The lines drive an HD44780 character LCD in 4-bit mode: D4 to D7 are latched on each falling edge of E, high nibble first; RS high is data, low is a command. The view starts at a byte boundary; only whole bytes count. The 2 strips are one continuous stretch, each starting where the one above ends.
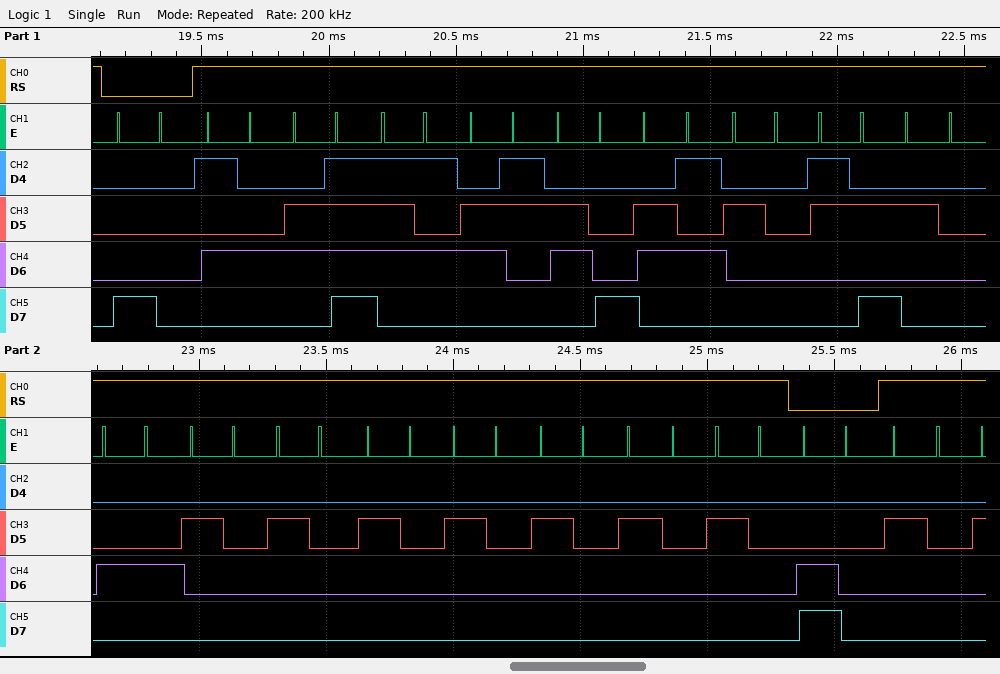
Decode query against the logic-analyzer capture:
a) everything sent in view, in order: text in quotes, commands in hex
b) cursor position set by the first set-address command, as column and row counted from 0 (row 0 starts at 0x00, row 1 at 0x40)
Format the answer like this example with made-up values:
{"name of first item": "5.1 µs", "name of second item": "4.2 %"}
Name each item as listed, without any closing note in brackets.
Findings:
{"everything sent in view, in order: text in quotes, commands in hex": "0x80 \"Touche : D       \" 0xC0 \" \"", "cursor position set by the first set-address command, as column and row counted from 0": "column 0, row 0"}
